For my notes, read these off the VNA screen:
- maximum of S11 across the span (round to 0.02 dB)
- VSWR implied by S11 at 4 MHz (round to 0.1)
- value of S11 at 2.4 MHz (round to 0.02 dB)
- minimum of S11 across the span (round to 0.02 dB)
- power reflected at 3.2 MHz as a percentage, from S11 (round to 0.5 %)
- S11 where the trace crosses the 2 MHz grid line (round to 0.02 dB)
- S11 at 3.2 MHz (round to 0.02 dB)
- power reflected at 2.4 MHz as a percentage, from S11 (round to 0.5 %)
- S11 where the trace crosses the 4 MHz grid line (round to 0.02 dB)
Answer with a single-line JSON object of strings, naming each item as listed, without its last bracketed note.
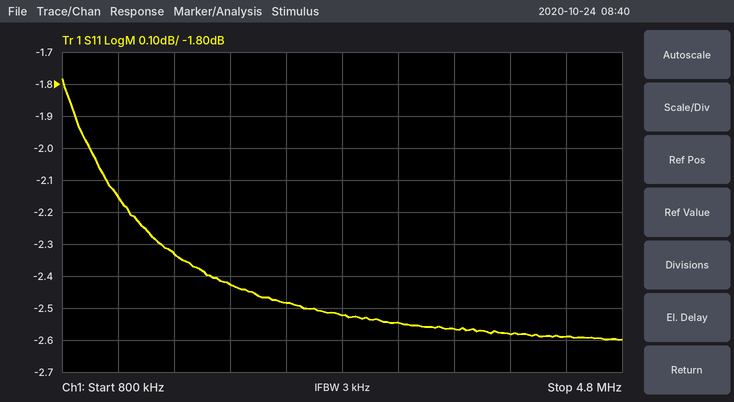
{"maximum of S11 across the span": "-1.78 dB", "VSWR implied by S11 at 4 MHz": "6.8", "value of S11 at 2.4 MHz": "-2.48 dB", "minimum of S11 across the span": "-2.60 dB", "power reflected at 3.2 MHz as a percentage, from S11": "55.5 %", "S11 where the trace crosses the 2 MHz grid line": "-2.42 dB", "S11 at 3.2 MHz": "-2.54 dB", "power reflected at 2.4 MHz as a percentage, from S11": "56.5 %", "S11 where the trace crosses the 4 MHz grid line": "-2.58 dB"}
